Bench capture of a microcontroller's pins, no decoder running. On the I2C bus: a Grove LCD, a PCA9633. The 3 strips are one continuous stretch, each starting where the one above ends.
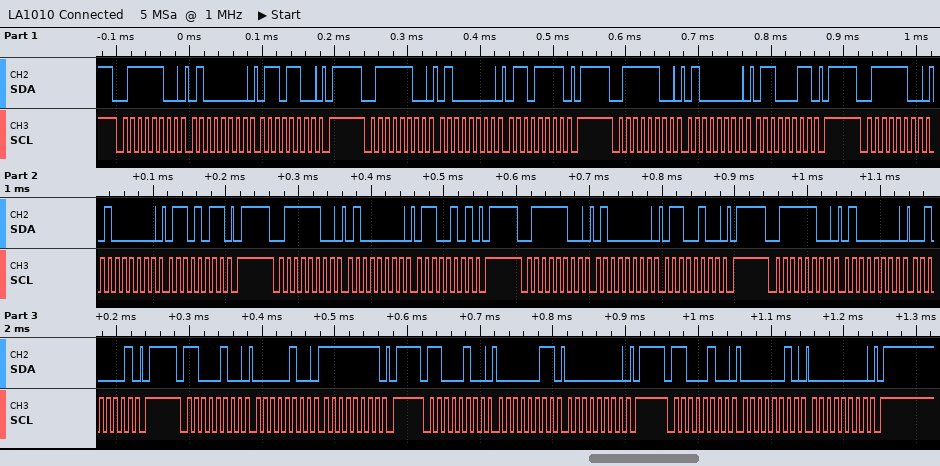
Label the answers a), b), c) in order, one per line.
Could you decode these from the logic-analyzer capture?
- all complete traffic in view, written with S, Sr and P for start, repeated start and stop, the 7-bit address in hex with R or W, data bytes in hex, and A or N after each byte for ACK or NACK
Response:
a) S 3EW A 40 A 6C A P S 3EW A 40 A 6F A P S 3EW A 40 A 63 A P S 3EW A 40 A 6B A P S 3EW A 40 A 65 A P S 3EW A 40 A 64 A P S 3EW A 40 A 21 A P S 62W A 04 A FF A P S 62W A 03 A 00 A P S 62W A 02 A 00 A P
